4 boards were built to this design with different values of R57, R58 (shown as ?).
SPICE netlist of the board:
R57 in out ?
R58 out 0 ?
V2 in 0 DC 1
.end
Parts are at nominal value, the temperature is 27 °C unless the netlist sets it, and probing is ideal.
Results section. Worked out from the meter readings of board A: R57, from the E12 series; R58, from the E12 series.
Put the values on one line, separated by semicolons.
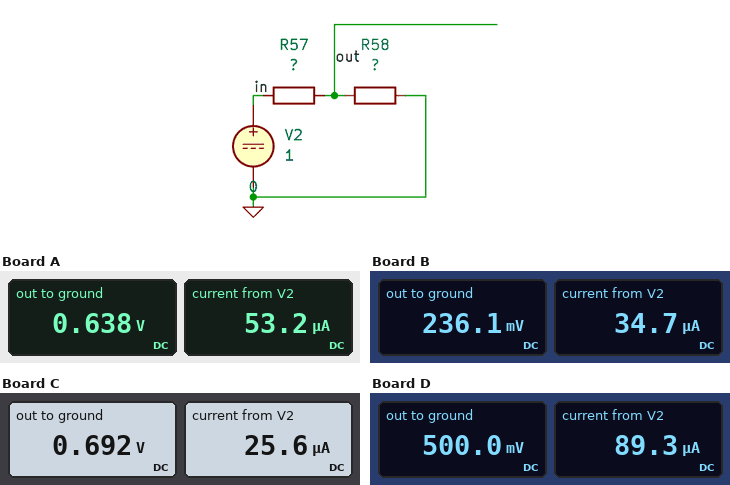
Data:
6.8 kΩ; 12 kΩ
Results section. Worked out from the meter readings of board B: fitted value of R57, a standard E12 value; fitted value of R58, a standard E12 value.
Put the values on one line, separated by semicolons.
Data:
22 kΩ; 6.8 kΩ
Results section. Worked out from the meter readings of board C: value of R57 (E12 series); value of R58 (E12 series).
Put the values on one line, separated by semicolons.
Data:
12 kΩ; 27 kΩ
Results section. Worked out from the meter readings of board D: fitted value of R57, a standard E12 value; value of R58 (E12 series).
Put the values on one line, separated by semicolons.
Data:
5.6 kΩ; 5.6 kΩ
